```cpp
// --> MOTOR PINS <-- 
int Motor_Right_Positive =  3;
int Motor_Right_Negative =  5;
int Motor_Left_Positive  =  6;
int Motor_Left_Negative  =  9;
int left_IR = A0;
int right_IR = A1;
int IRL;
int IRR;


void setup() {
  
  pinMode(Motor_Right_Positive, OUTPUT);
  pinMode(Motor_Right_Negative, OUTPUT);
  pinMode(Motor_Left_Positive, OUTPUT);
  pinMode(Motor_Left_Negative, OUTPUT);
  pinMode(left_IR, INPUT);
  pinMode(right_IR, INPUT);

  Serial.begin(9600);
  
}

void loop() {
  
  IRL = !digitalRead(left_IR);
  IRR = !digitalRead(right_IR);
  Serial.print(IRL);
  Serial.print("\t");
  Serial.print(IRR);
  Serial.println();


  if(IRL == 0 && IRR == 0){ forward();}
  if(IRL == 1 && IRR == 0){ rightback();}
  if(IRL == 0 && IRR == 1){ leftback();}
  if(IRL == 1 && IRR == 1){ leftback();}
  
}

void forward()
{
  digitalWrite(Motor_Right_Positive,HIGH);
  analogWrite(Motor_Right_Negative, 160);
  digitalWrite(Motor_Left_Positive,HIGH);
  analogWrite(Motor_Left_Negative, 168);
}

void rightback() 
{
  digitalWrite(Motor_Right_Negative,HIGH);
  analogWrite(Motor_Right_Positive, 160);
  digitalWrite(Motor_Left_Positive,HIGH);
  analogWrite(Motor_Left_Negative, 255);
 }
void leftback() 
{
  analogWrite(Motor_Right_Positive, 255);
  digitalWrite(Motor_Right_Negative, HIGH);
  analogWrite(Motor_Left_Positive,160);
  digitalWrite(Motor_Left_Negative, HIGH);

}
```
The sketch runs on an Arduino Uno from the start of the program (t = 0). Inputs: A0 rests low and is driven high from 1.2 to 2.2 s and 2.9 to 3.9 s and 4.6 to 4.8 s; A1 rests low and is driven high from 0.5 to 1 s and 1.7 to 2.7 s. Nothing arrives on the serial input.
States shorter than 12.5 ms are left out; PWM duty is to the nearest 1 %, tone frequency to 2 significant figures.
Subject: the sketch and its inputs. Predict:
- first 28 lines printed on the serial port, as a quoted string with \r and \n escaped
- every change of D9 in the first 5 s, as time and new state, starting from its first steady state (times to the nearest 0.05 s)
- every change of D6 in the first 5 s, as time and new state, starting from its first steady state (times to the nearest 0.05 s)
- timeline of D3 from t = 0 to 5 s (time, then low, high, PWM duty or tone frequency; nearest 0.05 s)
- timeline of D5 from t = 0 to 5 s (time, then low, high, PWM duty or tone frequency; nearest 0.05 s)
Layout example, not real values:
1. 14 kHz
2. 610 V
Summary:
1. "1\t1\r\n1\t1\r\n1\t1\r\n1\t1\r\n1\t1\r\n1\t1\r\n1\t1\r\n1\t1\r\n1\t1\r\n1\t1\r\n1\t1\r\n1\t1\r\n1\t1\r\n1\t1\r\n1\t1\r\n1\t1\r\n1\t1\r\n1\t1\r\n1\t1\r\n1\t1\r\n1\t1\r\n1\t1\r\n1\t1\r\n1\t1\r\n1\t1\r\n1\t1\r\n1\t1\r\n1\t1\r\n"
2. 0 s high; 1.7 s PWM 66 %; 2.2 s high
3. 0 s PWM 63 %; 0.5 s high; 1 s PWM 63 %; 1.7 s high; 2.7 s PWM 63 %
4. 0 s high; 0.5 s PWM 63 %; 1 s high; 2.2 s PWM 63 %; 2.7 s high
5. 0 s high; 1.7 s PWM 63 %; 2.2 s high
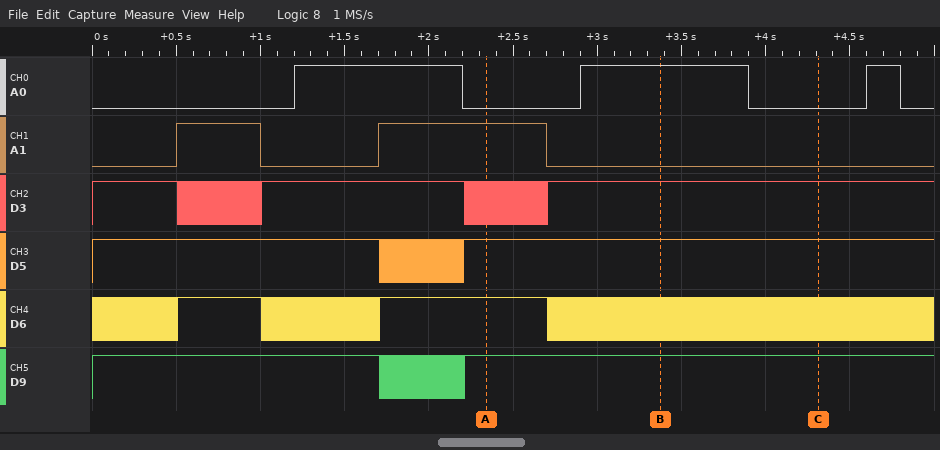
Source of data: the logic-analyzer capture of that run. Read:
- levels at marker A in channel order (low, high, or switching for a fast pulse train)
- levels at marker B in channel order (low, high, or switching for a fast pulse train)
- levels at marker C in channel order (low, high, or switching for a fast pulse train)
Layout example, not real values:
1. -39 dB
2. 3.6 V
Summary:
1. A0 low, A1 high, D3 switching, D5 high, D6 high, D9 high
2. A0 high, A1 low, D3 high, D5 high, D6 switching, D9 high
3. A0 low, A1 low, D3 high, D5 high, D6 switching, D9 high
